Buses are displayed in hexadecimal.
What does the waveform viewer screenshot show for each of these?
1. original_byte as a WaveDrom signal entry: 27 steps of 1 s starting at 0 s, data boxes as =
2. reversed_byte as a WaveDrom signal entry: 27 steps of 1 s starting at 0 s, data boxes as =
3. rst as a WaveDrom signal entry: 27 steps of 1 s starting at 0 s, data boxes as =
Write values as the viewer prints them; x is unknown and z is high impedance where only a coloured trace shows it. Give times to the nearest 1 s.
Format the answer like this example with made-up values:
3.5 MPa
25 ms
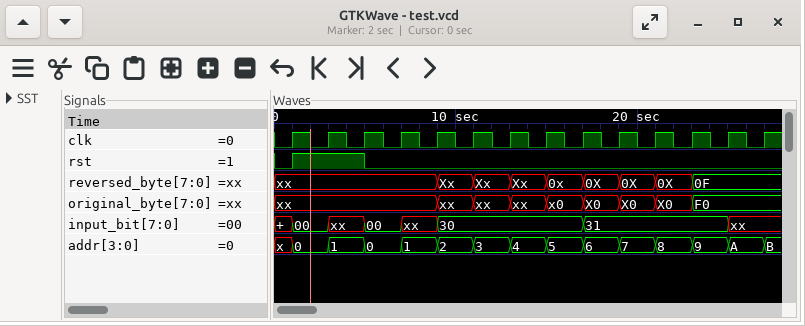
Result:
{name: 'original_byte', wave: 'x........=.=.=.=.=.=.=.=...', data: 'xx xx xx x0 X0 X0 X0 F0'}
{name: 'reversed_byte', wave: 'x........=.=.=.=.=.=.=.=...', data: 'Xx Xx Xx 0x 0X 0X 0X 0F'}
{name: 'rst', wave: '01...0.....................'}
